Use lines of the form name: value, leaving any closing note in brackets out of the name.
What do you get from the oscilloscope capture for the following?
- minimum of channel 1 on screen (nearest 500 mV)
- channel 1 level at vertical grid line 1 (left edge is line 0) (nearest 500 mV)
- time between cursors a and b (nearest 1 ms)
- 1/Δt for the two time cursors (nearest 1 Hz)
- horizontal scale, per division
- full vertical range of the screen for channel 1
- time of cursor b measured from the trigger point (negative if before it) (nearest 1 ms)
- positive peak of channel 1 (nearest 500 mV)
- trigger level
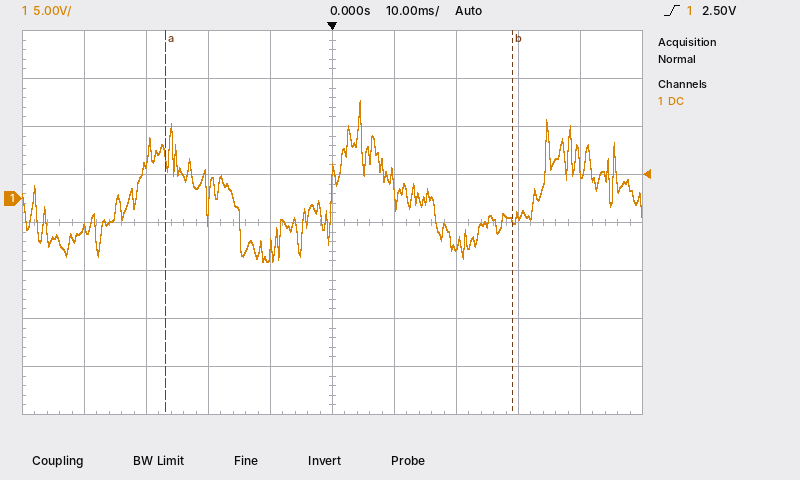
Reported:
minimum of channel 1 on screen: -6.5 V
channel 1 level at vertical grid line 1 (left edge is line 0): -3.0 V
time between cursors a and b: 56 ms
1/Δt for the two time cursors: 18 Hz
horizontal scale, per division: 10 ms
full vertical range of the screen for channel 1: 40 V
time of cursor b measured from the trigger point (negative if before it): +29 ms
positive peak of channel 1: 10.0 V
trigger level: 2.50 V
